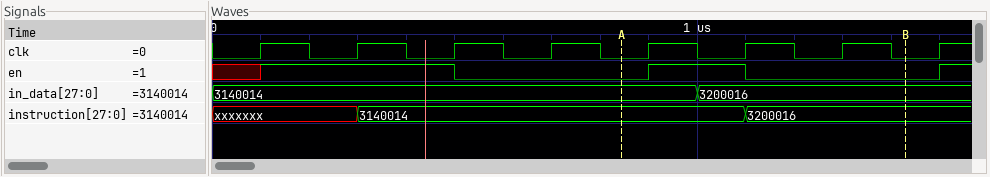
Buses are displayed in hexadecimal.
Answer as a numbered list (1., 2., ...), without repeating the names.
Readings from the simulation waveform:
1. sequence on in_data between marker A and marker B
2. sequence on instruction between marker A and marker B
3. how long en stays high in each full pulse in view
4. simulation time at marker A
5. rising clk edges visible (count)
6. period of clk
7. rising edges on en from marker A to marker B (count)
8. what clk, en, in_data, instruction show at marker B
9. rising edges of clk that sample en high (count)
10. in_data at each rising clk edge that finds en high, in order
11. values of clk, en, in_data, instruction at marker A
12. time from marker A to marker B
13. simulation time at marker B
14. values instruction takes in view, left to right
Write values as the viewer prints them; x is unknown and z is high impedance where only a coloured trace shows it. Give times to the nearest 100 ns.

1. 3140014, 3200016
2. 3140014, 3200016
3. 200 ns
4. 800 ns
5. 8
6. 200 ns
7. 1
8. clk=0, en=0, in_data=3200016, instruction=3200016
9. 3
10. 3140014, 3140014, 3200016
11. clk=0, en=0, in_data=3140014, instruction=3140014
12. 600 ns
13. 1400 ns
14. xxxxxxx, 3140014, 3200016
